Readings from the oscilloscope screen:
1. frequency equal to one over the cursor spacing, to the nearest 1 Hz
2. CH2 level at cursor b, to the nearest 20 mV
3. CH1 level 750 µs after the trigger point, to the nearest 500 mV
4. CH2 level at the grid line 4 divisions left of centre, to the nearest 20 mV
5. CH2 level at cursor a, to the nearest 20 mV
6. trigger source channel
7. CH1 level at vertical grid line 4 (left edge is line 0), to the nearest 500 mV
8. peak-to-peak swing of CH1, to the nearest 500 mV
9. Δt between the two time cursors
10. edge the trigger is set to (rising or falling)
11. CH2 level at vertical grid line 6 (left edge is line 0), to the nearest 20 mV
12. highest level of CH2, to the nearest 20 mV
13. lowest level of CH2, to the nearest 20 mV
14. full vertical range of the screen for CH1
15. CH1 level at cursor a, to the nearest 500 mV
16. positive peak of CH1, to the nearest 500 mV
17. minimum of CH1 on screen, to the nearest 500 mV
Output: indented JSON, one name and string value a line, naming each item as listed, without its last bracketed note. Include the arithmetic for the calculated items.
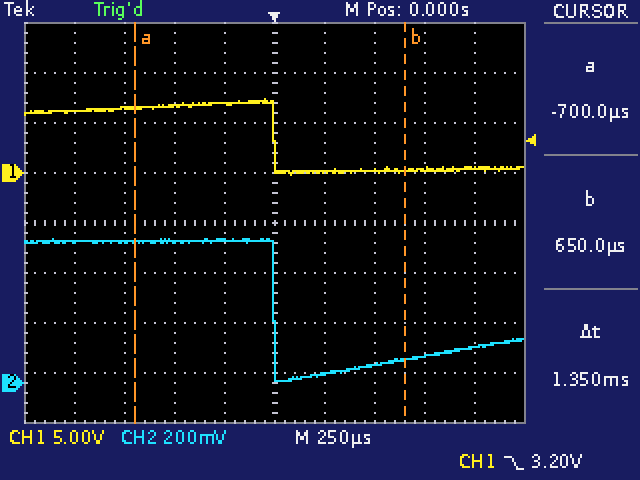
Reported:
{
  "frequency equal to one over the cursor spacing, to the nearest 1 Hz": "1 / 1.35 ms ≈ 741 Hz",
  "CH2 level at cursor b, to the nearest 20 mV": "100 mV",
  "CH1 level 750 µs after the trigger point, to the nearest 500 mV": "500 mV",
  "CH2 level at the grid line 4 divisions left of centre, to the nearest 20 mV": "560 mV",
  "CH2 level at cursor a, to the nearest 20 mV": "560 mV",
  "trigger source channel": "CH1",
  "CH1 level at vertical grid line 4 (left edge is line 0), to the nearest 500 mV": "7.0 V",
  "peak-to-peak swing of CH1, to the nearest 500 mV": "7.5 V − (0.0 V) = 7.5 V",
  "Δt between the two time cursors": "1.35 ms",
  "edge the trigger is set to": "falling",
  "CH2 level at vertical grid line 6 (left edge is line 0), to the nearest 20 mV": "40 mV",
  "highest level of CH2, to the nearest 20 mV": "580 mV",
  "lowest level of CH2, to the nearest 20 mV": "0 mV",
  "full vertical range of the screen for CH1": "40 V",
  "CH1 level at cursor a, to the nearest 500 mV": "6.5 V",
  "positive peak of CH1, to the nearest 500 mV": "7.5 V",
  "minimum of CH1 on screen, to the nearest 500 mV": "0.0 V"
}
